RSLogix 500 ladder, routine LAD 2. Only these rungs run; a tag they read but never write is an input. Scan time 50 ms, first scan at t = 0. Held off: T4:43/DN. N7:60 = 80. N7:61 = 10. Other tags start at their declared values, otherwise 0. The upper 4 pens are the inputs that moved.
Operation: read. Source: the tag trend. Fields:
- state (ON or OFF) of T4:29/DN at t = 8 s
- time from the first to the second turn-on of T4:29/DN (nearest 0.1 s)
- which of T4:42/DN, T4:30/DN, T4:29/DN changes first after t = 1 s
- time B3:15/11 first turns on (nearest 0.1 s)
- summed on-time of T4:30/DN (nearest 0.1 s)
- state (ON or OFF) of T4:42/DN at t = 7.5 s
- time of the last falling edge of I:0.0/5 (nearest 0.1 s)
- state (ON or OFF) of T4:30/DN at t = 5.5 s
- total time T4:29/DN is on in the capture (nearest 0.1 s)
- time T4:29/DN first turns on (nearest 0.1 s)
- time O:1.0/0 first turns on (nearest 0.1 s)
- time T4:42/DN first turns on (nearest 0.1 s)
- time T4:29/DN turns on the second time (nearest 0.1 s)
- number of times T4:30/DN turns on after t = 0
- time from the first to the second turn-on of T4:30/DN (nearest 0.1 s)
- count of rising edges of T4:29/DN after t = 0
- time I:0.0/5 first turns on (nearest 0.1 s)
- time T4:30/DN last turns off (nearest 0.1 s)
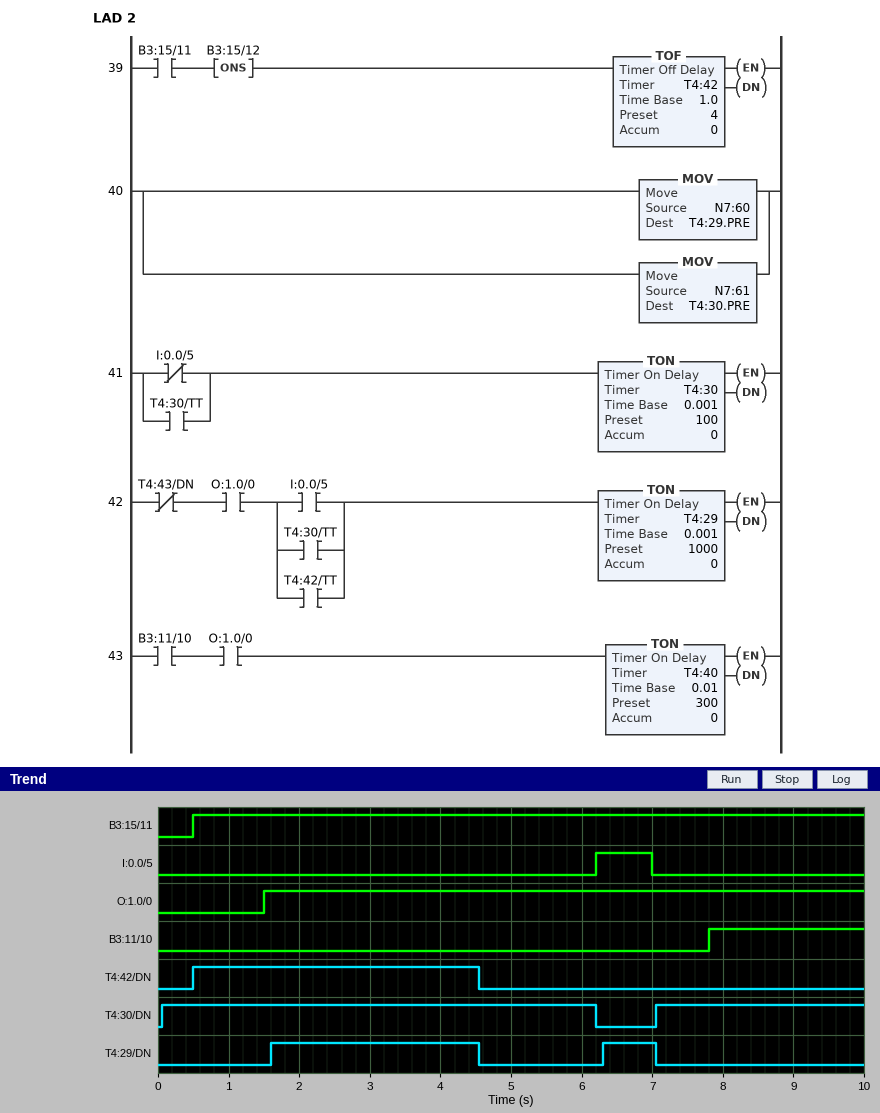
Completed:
OFF
4.7 s
T4:29/DN
0.5 s
9.1 s
OFF
7.0 s
ON
3.7 s
1.6 s
1.5 s
0.5 s
6.3 s
2
7.0 s
2
6.2 s
6.2 s
